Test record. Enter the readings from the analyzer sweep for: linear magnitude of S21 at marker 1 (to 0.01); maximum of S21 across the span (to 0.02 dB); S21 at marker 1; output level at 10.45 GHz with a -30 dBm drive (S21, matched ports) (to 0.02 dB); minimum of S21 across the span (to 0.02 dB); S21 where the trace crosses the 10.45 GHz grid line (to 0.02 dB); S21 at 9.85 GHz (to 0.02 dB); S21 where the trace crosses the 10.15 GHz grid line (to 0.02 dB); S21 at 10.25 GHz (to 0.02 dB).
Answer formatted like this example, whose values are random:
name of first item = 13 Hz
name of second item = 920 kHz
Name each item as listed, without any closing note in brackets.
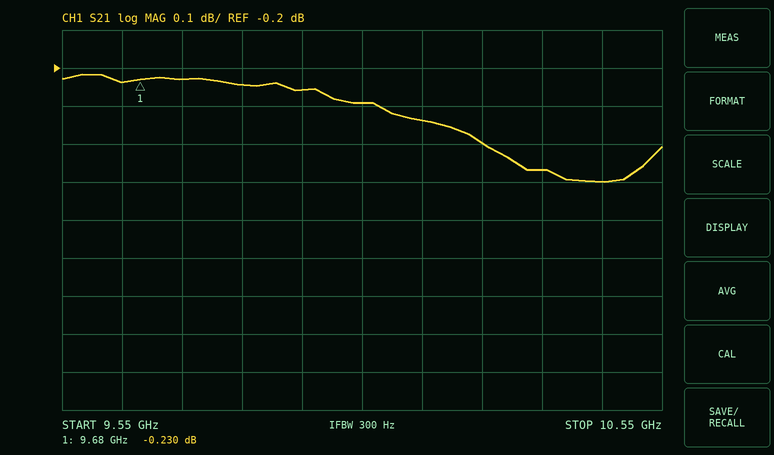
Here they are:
linear magnitude of S21 at marker 1 = 0.97
maximum of S21 across the span = -0.22 dB
S21 at marker 1 = -0.230 dB
output level at 10.45 GHz with a -30 dBm drive (S21, matched ports) = -30.50 dBm
minimum of S21 across the span = -0.50 dB
S21 where the trace crosses the 10.45 GHz grid line = -0.50 dB
S21 at 9.85 GHz = -0.24 dB
S21 where the trace crosses the 10.15 GHz grid line = -0.34 dB
S21 at 10.25 GHz = -0.40 dB
